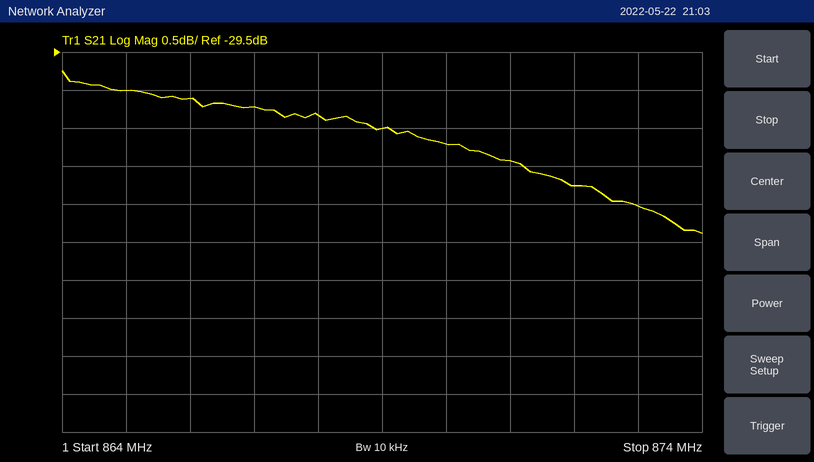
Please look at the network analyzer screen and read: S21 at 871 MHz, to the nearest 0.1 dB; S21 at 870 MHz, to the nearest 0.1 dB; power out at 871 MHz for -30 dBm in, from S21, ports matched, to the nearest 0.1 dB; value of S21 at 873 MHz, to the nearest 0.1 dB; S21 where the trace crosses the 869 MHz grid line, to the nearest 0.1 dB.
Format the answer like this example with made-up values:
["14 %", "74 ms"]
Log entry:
["-30.9 dB", "-30.7 dB", "-60.9 dBm", "-31.5 dB", "-30.5 dB"]
